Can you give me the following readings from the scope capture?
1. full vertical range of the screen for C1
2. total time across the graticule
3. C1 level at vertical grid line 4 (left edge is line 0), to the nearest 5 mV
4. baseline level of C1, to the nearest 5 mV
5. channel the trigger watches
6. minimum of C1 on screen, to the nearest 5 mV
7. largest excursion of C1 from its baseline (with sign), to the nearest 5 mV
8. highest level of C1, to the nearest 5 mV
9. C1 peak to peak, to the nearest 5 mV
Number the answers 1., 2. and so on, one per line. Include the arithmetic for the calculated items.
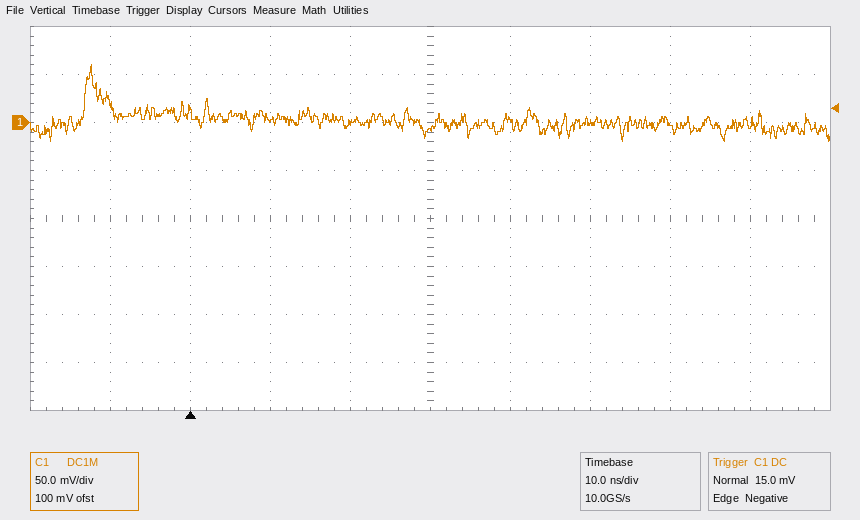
1. 400 mV
2. 100 ns
3. 0 mV
4. 0 mV
5. C1
6. -20 mV
7. 60 mV − (0 mV) = +60 mV
8. 60 mV
9. 60 mV − (-20 mV) = 80 mV
